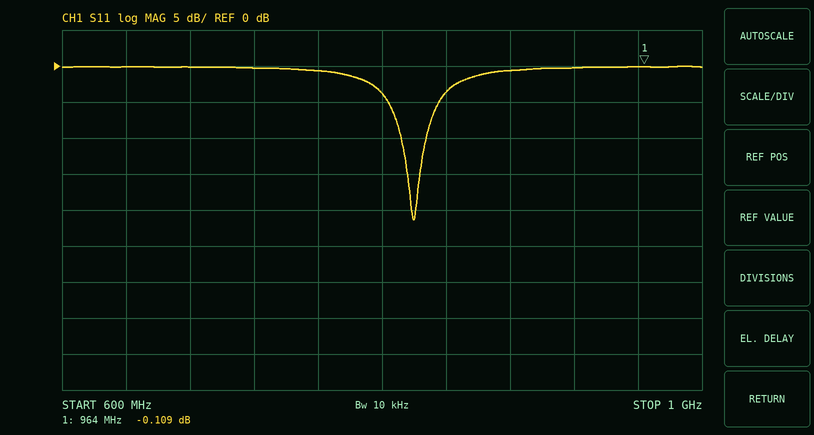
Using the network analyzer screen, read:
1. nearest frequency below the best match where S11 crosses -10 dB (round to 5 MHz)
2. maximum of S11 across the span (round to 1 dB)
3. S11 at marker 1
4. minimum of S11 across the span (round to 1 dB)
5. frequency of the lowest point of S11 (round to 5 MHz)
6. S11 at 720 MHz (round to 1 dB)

810 MHz
0 dB
-0.109 dB
-21 dB
820 MHz
0 dB
